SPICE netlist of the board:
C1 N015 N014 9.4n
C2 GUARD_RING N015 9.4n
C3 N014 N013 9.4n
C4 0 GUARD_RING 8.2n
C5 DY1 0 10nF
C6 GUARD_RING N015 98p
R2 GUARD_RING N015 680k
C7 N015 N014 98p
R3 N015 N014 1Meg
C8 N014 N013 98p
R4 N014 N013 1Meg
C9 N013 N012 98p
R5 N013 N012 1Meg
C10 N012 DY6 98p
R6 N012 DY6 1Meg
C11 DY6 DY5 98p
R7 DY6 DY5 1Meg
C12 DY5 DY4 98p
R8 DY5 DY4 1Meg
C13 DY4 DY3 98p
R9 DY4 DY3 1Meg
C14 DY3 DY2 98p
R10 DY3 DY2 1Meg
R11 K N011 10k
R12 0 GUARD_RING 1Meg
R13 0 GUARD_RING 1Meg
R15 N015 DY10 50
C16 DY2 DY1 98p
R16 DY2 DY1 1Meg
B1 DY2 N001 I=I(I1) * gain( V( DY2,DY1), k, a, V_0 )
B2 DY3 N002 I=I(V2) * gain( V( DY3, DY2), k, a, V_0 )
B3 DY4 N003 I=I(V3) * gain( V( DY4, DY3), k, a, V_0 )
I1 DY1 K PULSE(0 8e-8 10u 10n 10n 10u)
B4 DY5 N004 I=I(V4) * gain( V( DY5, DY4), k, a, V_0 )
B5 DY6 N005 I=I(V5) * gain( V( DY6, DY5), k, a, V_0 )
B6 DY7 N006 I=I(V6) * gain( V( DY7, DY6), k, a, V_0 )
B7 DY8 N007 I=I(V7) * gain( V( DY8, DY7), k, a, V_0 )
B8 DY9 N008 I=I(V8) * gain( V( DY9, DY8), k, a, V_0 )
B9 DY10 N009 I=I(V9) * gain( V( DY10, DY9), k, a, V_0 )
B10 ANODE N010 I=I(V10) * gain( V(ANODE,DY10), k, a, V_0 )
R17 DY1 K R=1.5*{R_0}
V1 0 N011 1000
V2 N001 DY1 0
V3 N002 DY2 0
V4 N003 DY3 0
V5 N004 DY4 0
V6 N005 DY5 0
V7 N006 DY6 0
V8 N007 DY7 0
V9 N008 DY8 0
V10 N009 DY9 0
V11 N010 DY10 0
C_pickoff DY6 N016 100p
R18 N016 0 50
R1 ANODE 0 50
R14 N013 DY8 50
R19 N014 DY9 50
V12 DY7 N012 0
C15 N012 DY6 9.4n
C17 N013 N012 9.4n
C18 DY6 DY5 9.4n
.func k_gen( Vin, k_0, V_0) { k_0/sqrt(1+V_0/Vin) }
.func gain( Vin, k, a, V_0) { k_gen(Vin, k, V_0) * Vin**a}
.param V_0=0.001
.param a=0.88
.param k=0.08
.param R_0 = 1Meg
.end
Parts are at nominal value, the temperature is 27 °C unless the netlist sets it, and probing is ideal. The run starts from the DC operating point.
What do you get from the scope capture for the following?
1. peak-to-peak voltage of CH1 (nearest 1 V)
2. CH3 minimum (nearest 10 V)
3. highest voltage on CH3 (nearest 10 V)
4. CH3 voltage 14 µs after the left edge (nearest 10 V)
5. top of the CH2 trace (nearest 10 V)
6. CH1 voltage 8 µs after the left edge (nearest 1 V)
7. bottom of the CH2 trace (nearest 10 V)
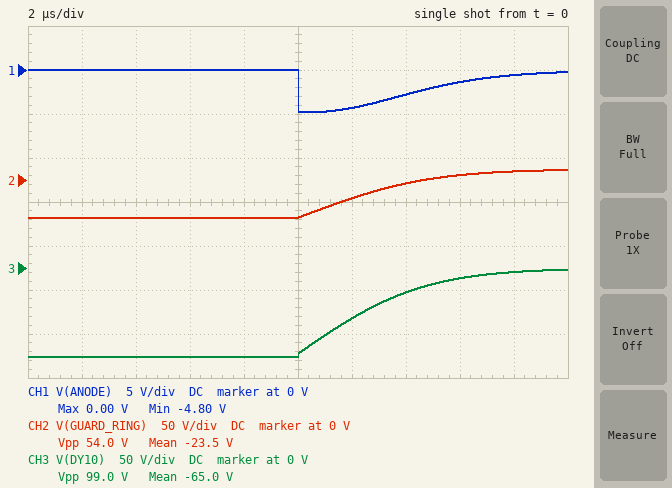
5 V
-100 V
0 V
-30 V
10 V
0 V
-40 V
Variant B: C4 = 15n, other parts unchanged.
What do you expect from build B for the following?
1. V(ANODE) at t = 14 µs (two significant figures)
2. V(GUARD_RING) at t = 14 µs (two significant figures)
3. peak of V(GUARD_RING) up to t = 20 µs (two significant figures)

-3.5 V
-20 V
-5.5 V
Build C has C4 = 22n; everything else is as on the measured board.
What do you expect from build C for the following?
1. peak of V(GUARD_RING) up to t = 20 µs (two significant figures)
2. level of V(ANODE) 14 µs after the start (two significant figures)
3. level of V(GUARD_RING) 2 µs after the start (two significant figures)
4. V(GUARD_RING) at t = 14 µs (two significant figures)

-15 V
-3.8 V
-43 V
-27 V
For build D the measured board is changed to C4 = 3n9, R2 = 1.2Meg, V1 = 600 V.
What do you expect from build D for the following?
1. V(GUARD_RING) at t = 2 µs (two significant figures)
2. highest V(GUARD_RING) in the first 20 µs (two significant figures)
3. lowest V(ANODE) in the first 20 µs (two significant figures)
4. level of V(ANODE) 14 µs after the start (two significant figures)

-25 V
-22 V
-54 mV
-53 mV
